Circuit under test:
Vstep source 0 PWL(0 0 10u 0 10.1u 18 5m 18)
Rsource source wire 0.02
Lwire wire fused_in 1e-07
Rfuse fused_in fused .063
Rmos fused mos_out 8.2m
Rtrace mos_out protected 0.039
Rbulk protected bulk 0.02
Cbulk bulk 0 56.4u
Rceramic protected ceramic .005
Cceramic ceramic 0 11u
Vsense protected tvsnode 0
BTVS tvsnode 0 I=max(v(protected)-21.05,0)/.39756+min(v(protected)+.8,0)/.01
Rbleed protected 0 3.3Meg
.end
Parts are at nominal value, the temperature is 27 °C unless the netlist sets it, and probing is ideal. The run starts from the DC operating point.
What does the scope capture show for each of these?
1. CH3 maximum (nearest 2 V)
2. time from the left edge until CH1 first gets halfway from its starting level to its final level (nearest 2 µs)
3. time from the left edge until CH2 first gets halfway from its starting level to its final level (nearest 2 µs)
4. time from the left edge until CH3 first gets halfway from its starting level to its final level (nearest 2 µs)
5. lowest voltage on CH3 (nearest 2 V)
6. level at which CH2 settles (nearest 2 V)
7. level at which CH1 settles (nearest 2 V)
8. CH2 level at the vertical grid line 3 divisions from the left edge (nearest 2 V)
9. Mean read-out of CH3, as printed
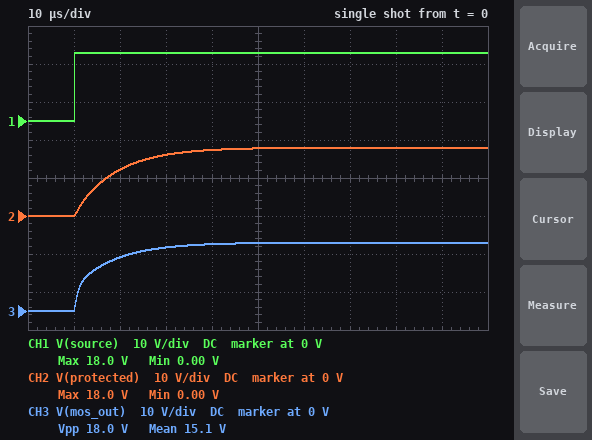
18 V
10 µs
16 µs
12 µs
0 V
18 V
18 V
16 V
15.1 V
